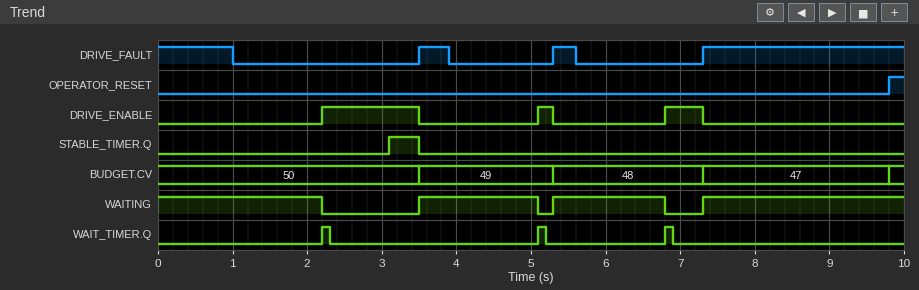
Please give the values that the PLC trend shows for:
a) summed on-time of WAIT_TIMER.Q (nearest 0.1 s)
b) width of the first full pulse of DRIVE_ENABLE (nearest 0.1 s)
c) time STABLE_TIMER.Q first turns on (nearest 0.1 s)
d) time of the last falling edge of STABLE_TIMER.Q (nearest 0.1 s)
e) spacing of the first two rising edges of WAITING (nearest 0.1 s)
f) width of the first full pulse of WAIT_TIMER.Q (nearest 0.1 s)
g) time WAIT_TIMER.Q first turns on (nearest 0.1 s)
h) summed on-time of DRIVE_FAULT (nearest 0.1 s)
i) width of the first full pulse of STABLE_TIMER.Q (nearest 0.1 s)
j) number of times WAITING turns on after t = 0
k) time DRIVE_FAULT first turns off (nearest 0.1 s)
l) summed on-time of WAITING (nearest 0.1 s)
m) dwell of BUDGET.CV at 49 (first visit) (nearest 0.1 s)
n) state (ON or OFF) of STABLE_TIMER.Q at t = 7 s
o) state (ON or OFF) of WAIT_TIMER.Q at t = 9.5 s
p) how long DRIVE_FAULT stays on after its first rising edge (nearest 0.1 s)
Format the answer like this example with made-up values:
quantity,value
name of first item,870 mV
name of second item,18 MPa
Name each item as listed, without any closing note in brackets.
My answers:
quantity,value
summed on-time of WAIT_TIMER.Q,0.3 s
width of the first full pulse of DRIVE_ENABLE,1.3 s
time STABLE_TIMER.Q first turns on,3.1 s
time of the last falling edge of STABLE_TIMER.Q,3.5 s
spacing of the first two rising edges of WAITING,1.8 s
width of the first full pulse of WAIT_TIMER.Q,0.1 s
time WAIT_TIMER.Q first turns on,2.2 s
summed on-time of DRIVE_FAULT,4.4 s
width of the first full pulse of STABLE_TIMER.Q,0.4 s
number of times WAITING turns on after t = 0,3
time DRIVE_FAULT first turns off,1.0 s
summed on-time of WAITING,8.0 s
dwell of BUDGET.CV at 49 (first visit),1.8 s
state (ON or OFF) of STABLE_TIMER.Q at t = 7 s,OFF
state (ON or OFF) of WAIT_TIMER.Q at t = 9.5 s,OFF
how long DRIVE_FAULT stays on after its first rising edge,0.4 s
